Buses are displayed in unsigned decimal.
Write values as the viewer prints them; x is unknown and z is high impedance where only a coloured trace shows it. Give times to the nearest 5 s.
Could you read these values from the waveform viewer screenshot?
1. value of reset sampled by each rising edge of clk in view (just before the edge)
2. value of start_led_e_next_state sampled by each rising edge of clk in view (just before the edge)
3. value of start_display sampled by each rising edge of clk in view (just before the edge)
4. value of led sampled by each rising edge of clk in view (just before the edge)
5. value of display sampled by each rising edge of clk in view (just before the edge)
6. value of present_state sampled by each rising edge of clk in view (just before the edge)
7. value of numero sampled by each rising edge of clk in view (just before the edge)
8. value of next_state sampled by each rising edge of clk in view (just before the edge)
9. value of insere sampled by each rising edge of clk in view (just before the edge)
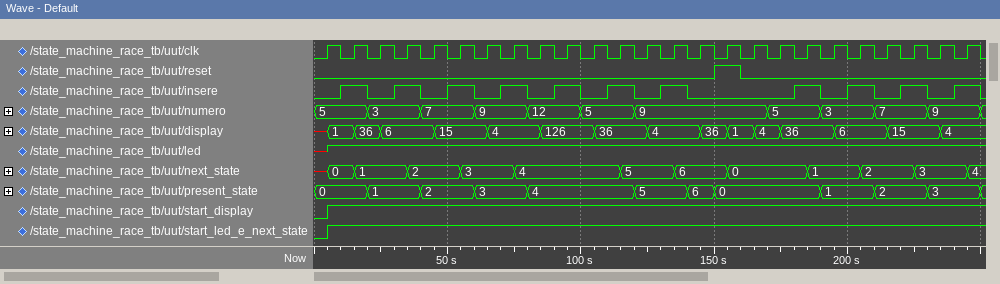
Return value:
0 0 0 0 0 0 0 0 0 0 0 0 0 0 0 1 0 0 0 0 0 0 0 0 0
0 1 1 1 1 1 1 1 1 1 1 1 1 1 1 1 1 1 1 1 1 1 1 1 1
0 1 1 1 1 1 1 1 1 1 1 1 1 1 1 1 1 1 1 1 1 1 1 1 1
x 1 1 1 1 1 1 1 1 1 1 1 1 1 1 1 1 1 1 1 1 1 1 1 1
x, 1, 36, 6, 6, 15, 15, 4, 4, 126, 126, 36, 36, 4, 4, 36, 1, 4, 36, 36, 6, 6, 15, 15, 4
0, 0, 1, 1, 2, 2, 3, 3, 4, 4, 4, 4, 5, 5, 6, 0, 0, 0, 0, 1, 1, 2, 2, 3, 3
5, 5, 3, 3, 7, 7, 9, 9, 12, 12, 5, 5, 9, 9, 9, 9, 9, 5, 5, 3, 3, 7, 7, 9, 9
x, 0, 1, 1, 2, 2, 3, 3, 4, 4, 4, 4, 5, 5, 6, 6, 0, 0, 0, 1, 1, 2, 2, 3, 3
0 1 0 1 0 1 0 1 0 1 0 1 0 1 0 0 0 0 1 0 1 0 1 0 1
